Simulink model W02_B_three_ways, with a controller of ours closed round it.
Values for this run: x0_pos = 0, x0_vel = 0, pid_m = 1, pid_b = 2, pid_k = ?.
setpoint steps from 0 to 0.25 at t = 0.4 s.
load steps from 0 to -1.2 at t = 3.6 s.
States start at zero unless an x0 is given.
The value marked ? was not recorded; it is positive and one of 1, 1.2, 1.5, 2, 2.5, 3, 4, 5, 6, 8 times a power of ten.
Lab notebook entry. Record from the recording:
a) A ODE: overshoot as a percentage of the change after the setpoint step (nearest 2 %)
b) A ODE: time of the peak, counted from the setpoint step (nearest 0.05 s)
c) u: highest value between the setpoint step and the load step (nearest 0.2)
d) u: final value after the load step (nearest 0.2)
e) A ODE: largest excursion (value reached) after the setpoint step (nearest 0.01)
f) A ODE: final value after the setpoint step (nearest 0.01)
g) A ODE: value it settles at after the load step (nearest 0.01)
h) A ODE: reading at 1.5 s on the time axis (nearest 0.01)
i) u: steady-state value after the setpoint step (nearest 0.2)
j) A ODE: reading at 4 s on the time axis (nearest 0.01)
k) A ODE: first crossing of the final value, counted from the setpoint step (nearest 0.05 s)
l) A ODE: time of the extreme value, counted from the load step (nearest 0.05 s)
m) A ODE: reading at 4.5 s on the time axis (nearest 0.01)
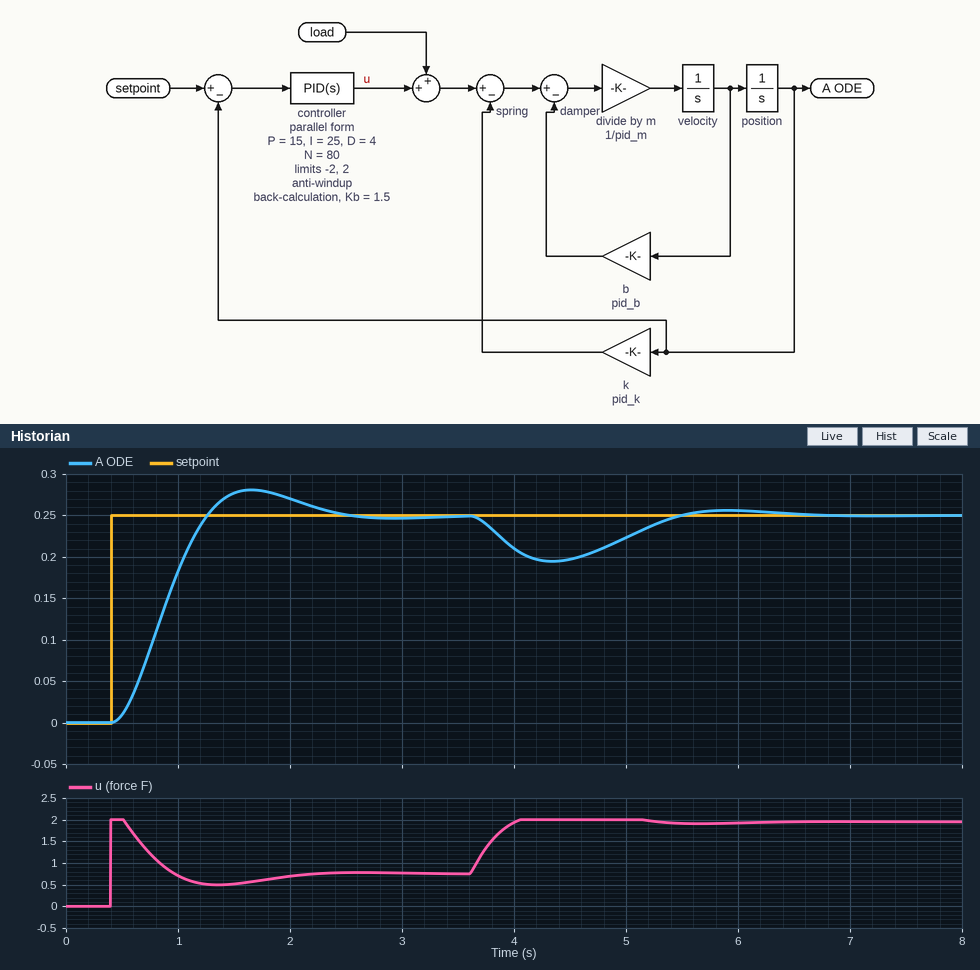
12 %
1.25 s
2.0
2.0
0.28
0.25
0.25
0.28
0.8
0.21
0.85 s
0.75 s
0.20
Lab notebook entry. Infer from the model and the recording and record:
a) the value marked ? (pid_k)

3
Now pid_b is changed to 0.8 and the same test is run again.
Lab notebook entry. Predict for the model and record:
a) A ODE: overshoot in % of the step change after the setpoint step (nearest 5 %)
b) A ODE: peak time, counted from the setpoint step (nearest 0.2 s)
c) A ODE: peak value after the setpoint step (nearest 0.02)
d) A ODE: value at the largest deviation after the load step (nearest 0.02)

15 %
1.0 s
0.28
0.18
